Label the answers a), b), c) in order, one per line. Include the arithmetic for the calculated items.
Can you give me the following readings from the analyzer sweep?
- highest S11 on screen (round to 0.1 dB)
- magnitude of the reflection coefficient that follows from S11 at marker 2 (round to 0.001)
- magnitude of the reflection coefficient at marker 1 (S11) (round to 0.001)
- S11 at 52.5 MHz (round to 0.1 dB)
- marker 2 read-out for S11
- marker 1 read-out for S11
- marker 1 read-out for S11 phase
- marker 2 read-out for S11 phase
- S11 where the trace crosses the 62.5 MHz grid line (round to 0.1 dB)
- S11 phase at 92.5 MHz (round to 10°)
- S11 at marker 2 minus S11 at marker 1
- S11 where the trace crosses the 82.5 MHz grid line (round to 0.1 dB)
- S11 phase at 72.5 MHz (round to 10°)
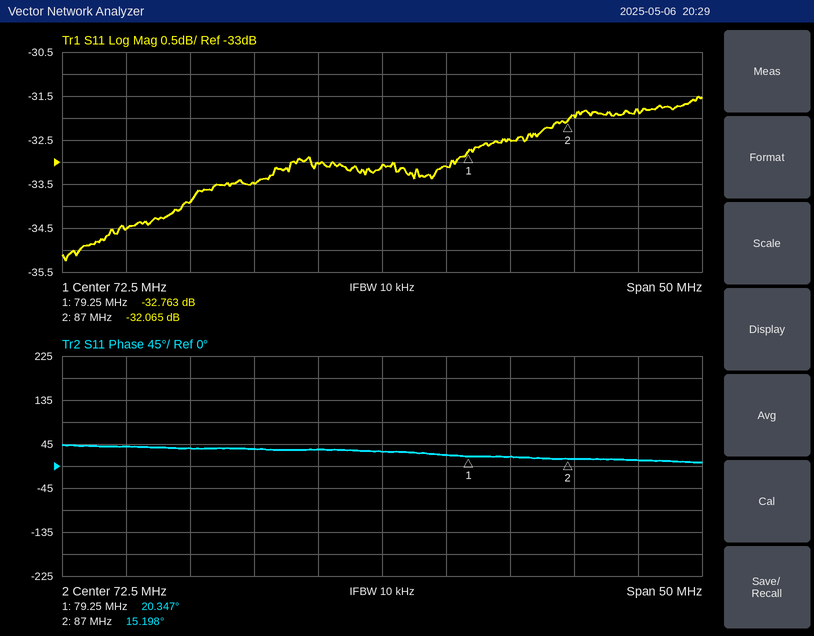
a) -31.5 dB
b) 10^(-32.065/20) ≈ 0.025
c) 10^(-32.763/20) ≈ 0.023
d) -34.5 dB
e) -32.065 dB
f) -32.763 dB
g) 20.347°
h) 15.198°
i) -33.5 dB
j) 10°
k) -32.065 − (-32.763) = 0.698 dB
l) -32.5 dB
m) 30°
